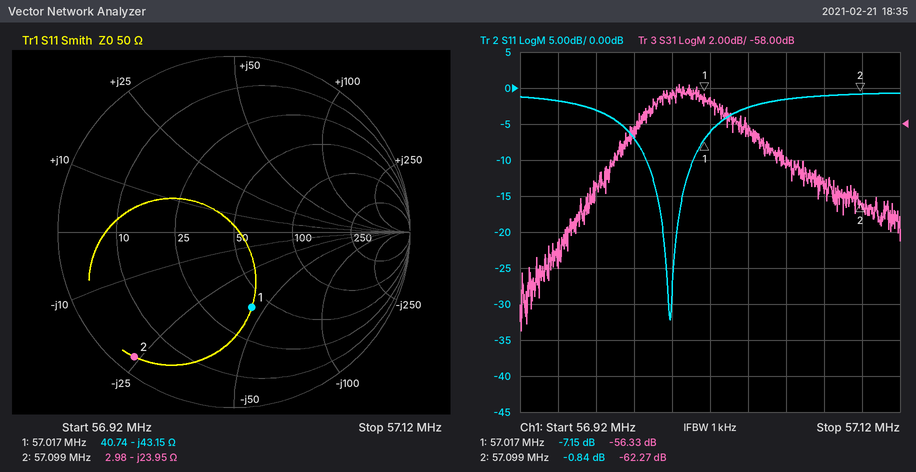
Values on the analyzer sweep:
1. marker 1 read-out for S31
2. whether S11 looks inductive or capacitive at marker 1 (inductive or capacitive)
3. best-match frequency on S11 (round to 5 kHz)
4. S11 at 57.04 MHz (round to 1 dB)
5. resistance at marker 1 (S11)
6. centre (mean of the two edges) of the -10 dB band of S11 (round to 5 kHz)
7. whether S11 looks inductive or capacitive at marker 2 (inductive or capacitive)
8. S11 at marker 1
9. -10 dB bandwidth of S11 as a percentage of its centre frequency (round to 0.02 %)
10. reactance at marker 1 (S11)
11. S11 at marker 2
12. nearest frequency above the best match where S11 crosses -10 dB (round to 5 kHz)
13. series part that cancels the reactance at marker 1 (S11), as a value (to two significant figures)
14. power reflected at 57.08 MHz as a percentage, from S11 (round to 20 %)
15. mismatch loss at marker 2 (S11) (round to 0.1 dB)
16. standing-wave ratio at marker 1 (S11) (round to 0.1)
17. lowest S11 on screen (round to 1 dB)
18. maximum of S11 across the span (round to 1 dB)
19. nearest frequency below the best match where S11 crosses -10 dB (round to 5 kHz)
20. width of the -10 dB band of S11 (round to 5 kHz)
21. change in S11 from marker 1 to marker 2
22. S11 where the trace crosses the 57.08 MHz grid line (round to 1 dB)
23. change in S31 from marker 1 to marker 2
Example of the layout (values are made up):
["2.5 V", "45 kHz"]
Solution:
["-56.33 dB", "capacitive", "57.000 MHz", "-3 dB", "40.74 Ω", "57.000 MHz", "capacitive", "-7.15 dB", "0.04 %", "-43.15 Ω", "-0.84 dB", "57.010 MHz", "120 nH", "80 %", "7.5 dB", "2.6", "-32 dB", "-1 dB", "56.985 MHz", "25 kHz", "6.31 dB", "-1 dB", "-5.94 dB"]
